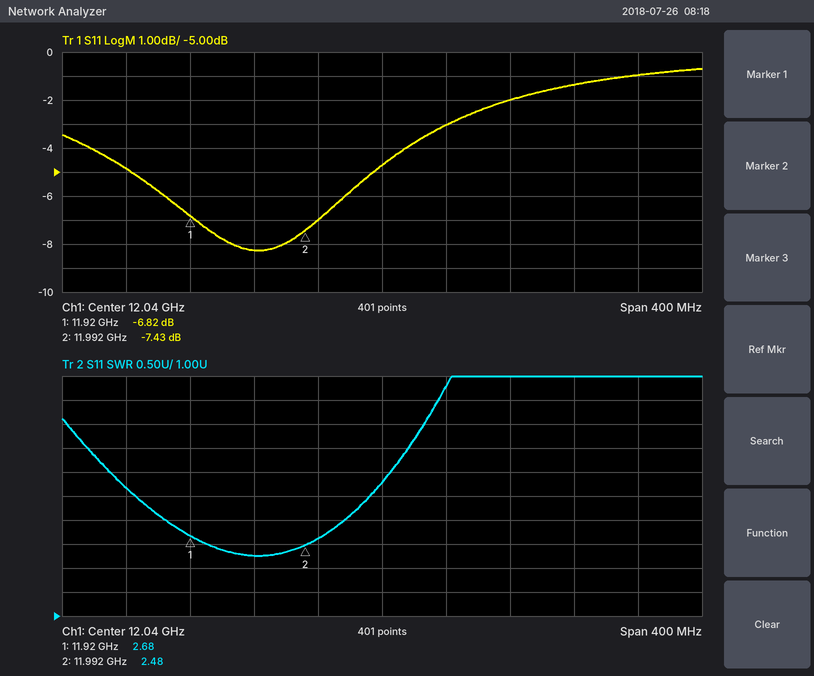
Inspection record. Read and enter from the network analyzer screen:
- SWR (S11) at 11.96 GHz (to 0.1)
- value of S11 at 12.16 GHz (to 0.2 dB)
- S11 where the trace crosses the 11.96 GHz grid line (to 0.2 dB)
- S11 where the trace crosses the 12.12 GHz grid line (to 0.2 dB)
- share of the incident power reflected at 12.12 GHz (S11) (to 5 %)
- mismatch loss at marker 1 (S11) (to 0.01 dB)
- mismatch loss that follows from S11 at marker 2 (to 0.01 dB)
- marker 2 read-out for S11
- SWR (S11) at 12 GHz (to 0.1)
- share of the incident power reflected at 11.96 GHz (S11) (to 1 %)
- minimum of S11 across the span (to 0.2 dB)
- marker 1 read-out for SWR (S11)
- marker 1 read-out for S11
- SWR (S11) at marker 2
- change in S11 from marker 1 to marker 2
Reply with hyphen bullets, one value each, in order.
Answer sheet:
- 2.3
- -1.4 dB
- -8.2 dB
- -2.0 dB
- 65 %
- 1.01 dB
- 0.87 dB
- -7.43 dB
- 2.6
- 15 %
- -8.2 dB
- 2.68
- -6.82 dB
- 2.48
- -0.61 dB
